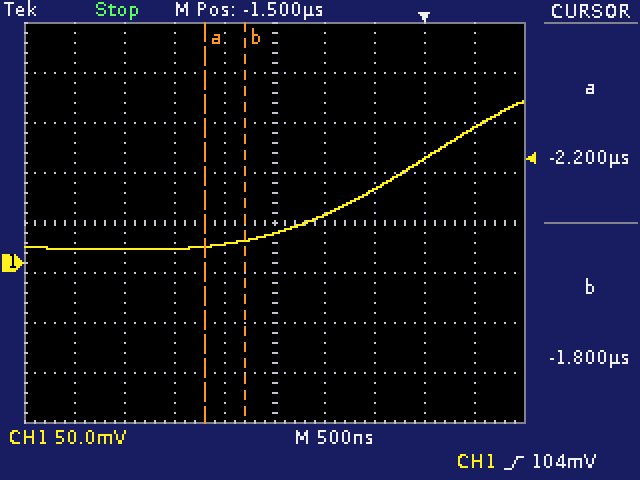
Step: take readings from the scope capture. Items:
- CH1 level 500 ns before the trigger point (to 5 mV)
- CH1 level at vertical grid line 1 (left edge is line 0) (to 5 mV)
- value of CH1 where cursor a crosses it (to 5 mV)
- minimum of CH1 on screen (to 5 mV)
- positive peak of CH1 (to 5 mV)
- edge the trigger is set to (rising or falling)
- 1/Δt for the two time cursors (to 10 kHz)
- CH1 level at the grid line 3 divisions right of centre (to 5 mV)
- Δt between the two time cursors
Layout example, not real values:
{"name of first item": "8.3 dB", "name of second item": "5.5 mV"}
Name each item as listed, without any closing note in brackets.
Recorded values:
{"CH1 level 500 ns before the trigger point": "75 mV", "CH1 level at vertical grid line 1 (left edge is line 0)": "15 mV", "value of CH1 where cursor a crosses it": "15 mV", "minimum of CH1 on screen": "15 mV", "positive peak of CH1": "160 mV", "edge the trigger is set to": "rising", "1/Δt for the two time cursors": "2.50 MHz", "CH1 level at the grid line 3 divisions right of centre": "105 mV", "Δt between the two time cursors": "400 ns"}
